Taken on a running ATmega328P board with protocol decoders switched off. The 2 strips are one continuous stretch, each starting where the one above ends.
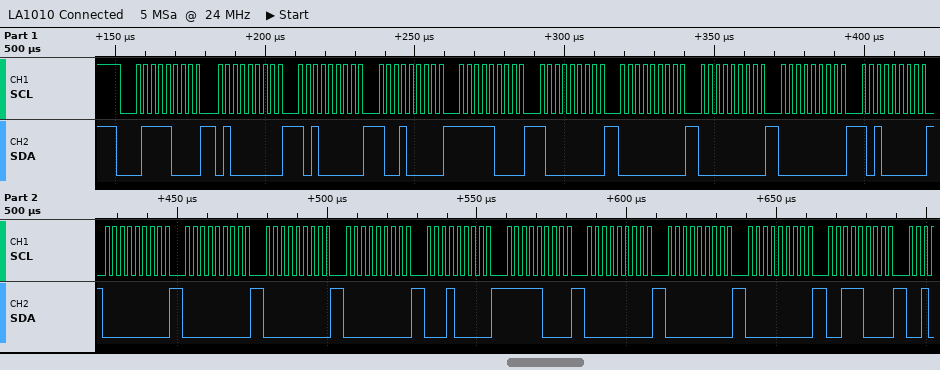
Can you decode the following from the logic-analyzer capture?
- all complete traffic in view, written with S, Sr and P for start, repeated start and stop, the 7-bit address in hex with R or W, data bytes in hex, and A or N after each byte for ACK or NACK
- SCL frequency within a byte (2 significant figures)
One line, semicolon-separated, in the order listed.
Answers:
S 3CW A 40 A A0 A 90 A F8 A 80 A 00 A 00 A 00 A A0 A 00 A 00 A 00 A 00 A 10 A F8 A 00 A 00 A 00 A 38 A; 400 kHz
